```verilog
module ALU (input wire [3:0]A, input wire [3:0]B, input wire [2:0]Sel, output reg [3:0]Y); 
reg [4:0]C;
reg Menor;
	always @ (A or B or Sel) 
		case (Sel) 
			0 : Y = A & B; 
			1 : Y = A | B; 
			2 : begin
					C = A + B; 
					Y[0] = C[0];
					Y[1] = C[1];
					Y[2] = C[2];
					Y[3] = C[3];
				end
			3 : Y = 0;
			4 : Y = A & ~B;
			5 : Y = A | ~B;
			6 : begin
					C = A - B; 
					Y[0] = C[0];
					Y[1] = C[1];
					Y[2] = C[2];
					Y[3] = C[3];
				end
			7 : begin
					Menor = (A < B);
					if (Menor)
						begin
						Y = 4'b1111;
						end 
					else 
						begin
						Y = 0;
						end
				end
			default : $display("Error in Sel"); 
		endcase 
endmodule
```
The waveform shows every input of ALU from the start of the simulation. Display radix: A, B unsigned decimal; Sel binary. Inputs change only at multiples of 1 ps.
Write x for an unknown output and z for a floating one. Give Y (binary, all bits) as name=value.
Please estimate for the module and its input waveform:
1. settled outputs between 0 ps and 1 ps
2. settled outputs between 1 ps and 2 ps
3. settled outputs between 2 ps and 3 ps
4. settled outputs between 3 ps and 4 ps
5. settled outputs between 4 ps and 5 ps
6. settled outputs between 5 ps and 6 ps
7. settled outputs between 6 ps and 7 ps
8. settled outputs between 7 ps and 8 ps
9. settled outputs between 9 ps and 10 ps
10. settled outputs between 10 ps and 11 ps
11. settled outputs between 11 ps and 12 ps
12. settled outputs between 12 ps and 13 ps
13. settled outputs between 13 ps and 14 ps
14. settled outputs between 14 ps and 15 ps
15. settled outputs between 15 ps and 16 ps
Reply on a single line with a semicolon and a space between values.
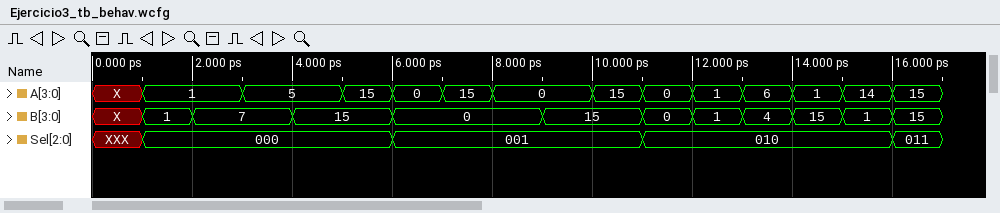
Y=x; Y=0001; Y=0001; Y=0101; Y=0101; Y=1111; Y=0000; Y=1111; Y=1111; Y=1111; Y=0000; Y=0010; Y=1010; Y=0000; Y=1111
